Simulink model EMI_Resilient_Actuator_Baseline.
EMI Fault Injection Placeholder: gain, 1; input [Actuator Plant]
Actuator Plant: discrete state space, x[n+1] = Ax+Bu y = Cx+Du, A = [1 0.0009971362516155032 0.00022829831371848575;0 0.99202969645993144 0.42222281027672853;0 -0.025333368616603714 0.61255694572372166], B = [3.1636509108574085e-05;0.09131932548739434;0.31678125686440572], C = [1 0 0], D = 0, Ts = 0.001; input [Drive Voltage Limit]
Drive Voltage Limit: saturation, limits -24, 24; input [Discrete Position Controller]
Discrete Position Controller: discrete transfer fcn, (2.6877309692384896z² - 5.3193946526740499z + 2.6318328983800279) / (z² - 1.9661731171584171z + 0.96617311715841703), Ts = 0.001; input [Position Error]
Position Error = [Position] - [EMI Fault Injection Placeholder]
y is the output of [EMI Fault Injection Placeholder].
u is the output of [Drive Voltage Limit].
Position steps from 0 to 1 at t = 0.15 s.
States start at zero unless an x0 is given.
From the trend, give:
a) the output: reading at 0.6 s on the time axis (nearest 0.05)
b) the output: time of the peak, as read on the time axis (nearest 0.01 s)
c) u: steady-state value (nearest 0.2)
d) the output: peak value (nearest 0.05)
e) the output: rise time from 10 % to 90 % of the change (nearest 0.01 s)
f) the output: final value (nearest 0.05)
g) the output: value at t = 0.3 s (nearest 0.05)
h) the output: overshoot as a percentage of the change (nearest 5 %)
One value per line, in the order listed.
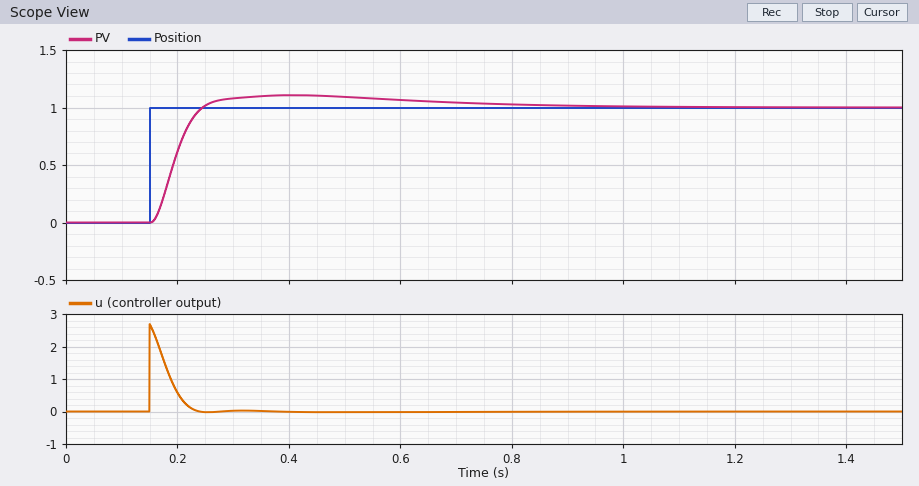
1.05
0.41 s
0.0
1.10
0.06 s
1.00
1.10
10 %
